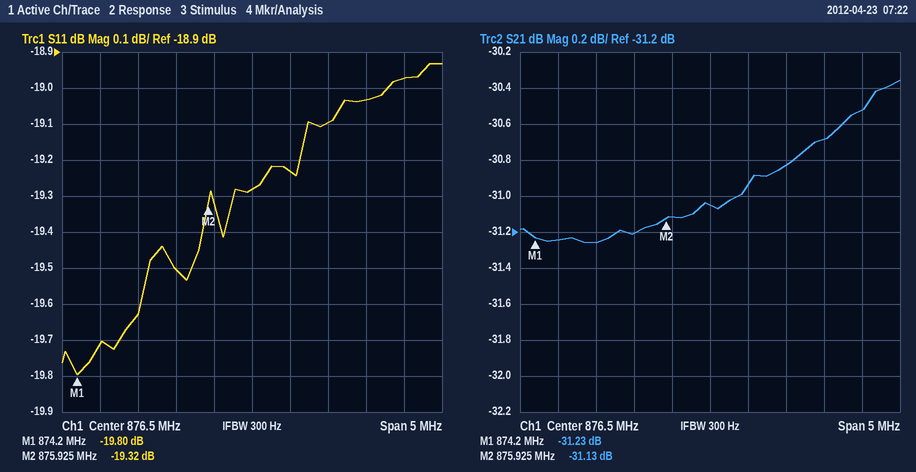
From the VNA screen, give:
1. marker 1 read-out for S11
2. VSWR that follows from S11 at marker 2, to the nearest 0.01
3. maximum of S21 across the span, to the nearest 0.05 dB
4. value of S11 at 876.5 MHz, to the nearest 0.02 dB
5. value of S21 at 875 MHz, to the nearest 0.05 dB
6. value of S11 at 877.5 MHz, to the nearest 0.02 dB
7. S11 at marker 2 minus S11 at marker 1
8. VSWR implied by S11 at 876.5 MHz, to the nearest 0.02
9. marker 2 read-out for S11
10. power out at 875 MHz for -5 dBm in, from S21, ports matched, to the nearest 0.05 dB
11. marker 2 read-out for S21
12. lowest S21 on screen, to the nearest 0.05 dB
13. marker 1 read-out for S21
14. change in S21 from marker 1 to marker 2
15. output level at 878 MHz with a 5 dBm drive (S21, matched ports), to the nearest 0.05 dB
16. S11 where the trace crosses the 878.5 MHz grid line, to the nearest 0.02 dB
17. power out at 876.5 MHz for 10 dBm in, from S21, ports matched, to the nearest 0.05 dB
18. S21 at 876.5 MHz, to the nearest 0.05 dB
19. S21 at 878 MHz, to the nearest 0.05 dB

-19.80 dB
1.24
-30.35 dB
-19.28 dB
-31.25 dB
-19.10 dB
0.48 dB
1.24
-19.32 dB
-36.25 dBm
-31.13 dB
-31.25 dB
-31.23 dB
0.10 dB
-25.70 dBm
-18.98 dB
-21.05 dBm
-31.05 dB
-30.70 dB
